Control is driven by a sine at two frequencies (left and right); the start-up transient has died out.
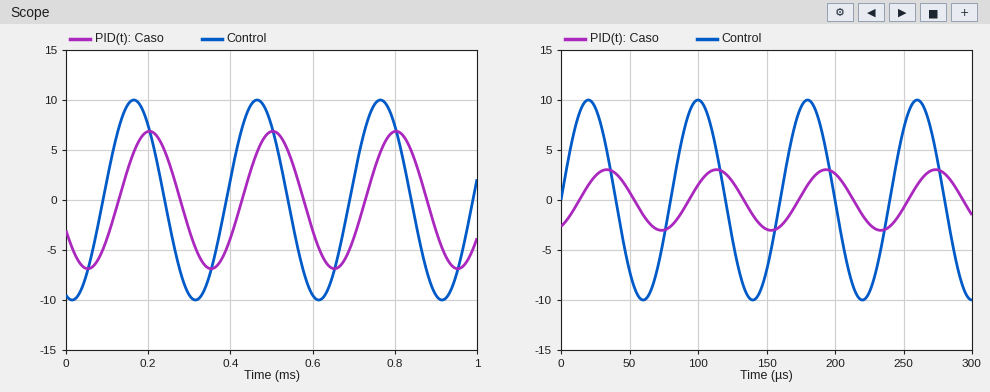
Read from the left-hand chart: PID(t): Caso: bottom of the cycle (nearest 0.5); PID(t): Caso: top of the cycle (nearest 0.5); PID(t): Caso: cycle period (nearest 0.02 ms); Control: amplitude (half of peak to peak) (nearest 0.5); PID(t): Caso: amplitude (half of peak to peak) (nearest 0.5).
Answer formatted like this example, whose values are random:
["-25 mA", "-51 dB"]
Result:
["-7.0", "7.0", "0.30 ms", "10.0", "7.0"]
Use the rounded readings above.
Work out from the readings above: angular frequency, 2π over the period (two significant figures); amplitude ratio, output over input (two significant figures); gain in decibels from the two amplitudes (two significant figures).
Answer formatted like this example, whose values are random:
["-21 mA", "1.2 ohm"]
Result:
["21 rad/ms", "0.70", "-3.1 dB"]
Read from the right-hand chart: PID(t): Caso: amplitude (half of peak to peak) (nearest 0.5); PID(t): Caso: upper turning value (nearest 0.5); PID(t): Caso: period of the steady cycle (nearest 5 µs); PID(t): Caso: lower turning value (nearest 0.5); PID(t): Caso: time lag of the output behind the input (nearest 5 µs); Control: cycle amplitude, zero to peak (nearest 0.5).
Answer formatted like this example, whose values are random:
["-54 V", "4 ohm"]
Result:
["3.0", "3.0", "80 µs", "-3.0", "15 µs", "10.0"]
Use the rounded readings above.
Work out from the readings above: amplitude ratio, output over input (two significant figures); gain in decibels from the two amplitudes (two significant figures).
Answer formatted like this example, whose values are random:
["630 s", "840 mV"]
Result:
["0.30", "-10 dB"]
